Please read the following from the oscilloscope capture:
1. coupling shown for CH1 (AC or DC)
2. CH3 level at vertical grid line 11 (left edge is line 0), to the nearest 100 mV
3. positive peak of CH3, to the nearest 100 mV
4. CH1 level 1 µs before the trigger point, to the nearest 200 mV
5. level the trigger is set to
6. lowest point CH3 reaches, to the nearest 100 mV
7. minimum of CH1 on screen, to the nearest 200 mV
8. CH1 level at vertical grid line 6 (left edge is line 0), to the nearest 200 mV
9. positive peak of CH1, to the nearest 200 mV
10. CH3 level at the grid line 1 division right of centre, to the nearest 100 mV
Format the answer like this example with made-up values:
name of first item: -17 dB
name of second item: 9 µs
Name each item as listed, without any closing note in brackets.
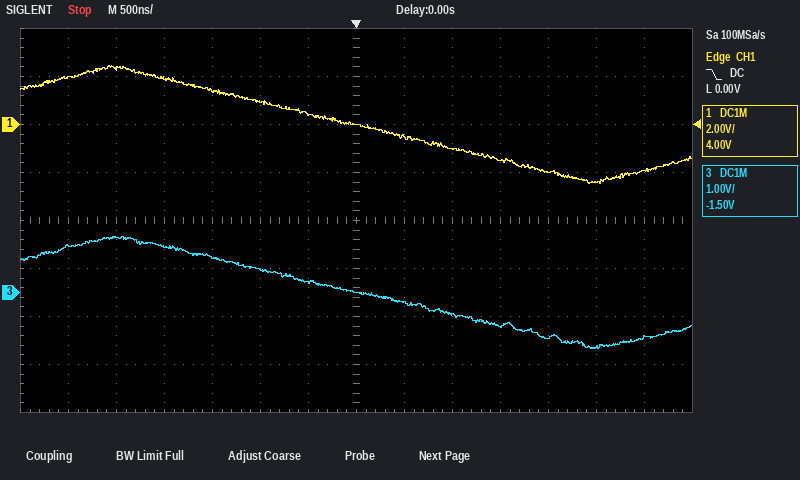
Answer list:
coupling shown for CH1: DC
CH3 level at vertical grid line 11 (left edge is line 0), to the nearest 100 mV: -900 mV
positive peak of CH3, to the nearest 100 mV: 1.2 V
CH1 level 1 µs before the trigger point, to the nearest 200 mV: 1.0 V
level the trigger is set to: 0.00 V
lowest point CH3 reaches, to the nearest 100 mV: -1.2 V
minimum of CH1 on screen, to the nearest 200 mV: -2.4 V
CH1 level at vertical grid line 6 (left edge is line 0), to the nearest 200 mV: 400 mV
positive peak of CH1, to the nearest 200 mV: 2.4 V
CH3 level at the grid line 1 division right of centre, to the nearest 100 mV: -200 mV
